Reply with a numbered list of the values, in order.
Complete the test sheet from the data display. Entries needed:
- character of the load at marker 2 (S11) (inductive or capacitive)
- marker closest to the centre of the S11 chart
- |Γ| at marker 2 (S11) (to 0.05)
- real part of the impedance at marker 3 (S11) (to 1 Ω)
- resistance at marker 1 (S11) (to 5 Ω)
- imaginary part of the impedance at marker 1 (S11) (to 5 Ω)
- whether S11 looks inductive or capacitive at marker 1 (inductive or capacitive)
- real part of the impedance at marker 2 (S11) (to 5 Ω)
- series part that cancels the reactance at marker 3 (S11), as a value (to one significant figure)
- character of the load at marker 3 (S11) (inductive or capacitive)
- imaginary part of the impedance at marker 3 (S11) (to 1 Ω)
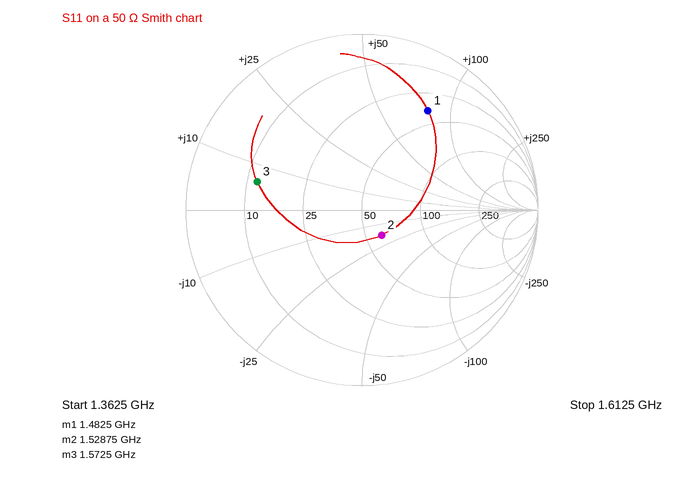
1. capacitive
2. marker 2
3. 0.20
4. 12 Ω
5. 40 Ω
6. +80 Ω
7. inductive
8. 60 Ω
9. 20 pF
10. inductive
11. +6 Ω
